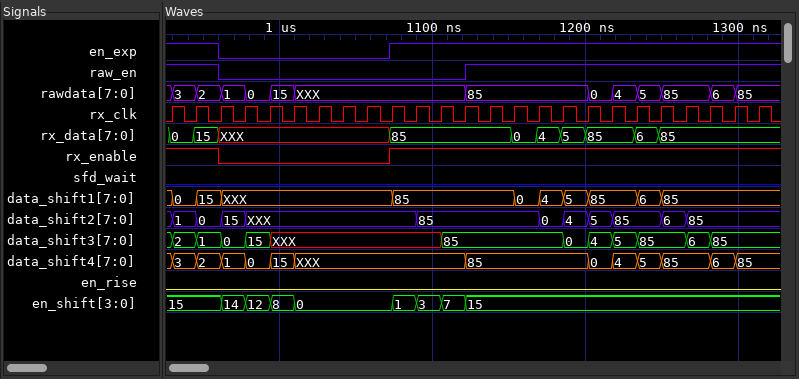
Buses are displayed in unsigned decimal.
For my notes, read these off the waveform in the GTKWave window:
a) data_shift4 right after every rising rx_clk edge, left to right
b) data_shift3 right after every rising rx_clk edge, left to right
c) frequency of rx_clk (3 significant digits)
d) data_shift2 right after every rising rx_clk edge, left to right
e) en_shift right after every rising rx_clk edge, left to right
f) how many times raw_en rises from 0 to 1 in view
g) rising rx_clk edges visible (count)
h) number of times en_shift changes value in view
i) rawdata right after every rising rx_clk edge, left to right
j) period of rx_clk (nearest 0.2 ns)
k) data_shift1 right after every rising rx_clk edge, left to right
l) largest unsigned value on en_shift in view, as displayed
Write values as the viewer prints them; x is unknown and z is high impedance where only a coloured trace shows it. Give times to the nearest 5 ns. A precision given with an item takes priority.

3, 2, 1, 0, 15, XXX, XXX, XXX, XXX, XXX, XXX, XXX, 85, 85, 85, 85, 85, 0, 4, 5, 85, 85, 6, 85, 85
2, 1, 0, 15, XXX, XXX, XXX, XXX, XXX, XXX, XXX, 85, 85, 85, 85, 85, 0, 4, 5, 85, 85, 6, 85, 85, 85
62.5 MHz
1, 0, 15, XXX, XXX, XXX, XXX, XXX, XXX, XXX, 85, 85, 85, 85, 85, 0, 4, 5, 85, 85, 6, 85, 85, 85, 85
15, 15, 14, 12, 8, 0, 0, 0, 0, 1, 3, 7, 15, 15, 15, 15, 15, 15, 15, 15, 15, 15, 15, 15, 15
1
25
8
3, 2, 1, 0, 15, XXX, XXX, XXX, XXX, XXX, XXX, XXX, 85, 85, 85, 85, 85, 0, 4, 5, 85, 85, 6, 85, 85
16 ns
0, 15, XXX, XXX, XXX, XXX, XXX, XXX, XXX, 85, 85, 85, 85, 85, 0, 4, 5, 85, 85, 6, 85, 85, 85, 85, 85
15
